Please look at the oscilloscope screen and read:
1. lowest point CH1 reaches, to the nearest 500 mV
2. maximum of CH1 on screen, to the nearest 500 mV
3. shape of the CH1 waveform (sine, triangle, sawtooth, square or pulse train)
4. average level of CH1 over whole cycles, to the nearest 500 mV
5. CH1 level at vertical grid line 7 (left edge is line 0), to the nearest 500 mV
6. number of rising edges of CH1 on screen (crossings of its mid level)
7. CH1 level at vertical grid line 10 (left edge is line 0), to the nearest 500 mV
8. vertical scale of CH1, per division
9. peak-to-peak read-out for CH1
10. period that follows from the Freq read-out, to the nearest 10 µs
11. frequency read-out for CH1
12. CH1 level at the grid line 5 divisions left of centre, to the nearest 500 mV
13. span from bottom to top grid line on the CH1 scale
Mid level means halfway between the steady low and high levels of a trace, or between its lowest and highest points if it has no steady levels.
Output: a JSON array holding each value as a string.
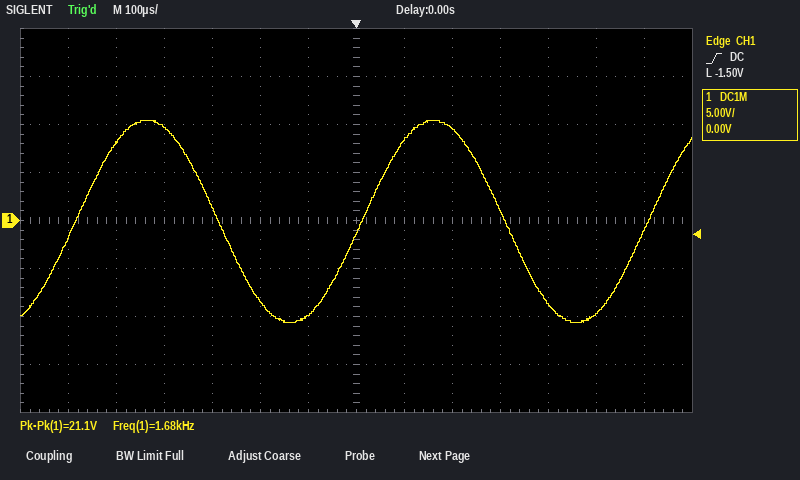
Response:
["-10.5 V", "10.5 V", "sine", "0.0 V", "-1.5 V", "3", "1.0 V", "5 V", "21.1 V", "600 µs", "1.68 kHz", "8.0 V", "40 V"]
